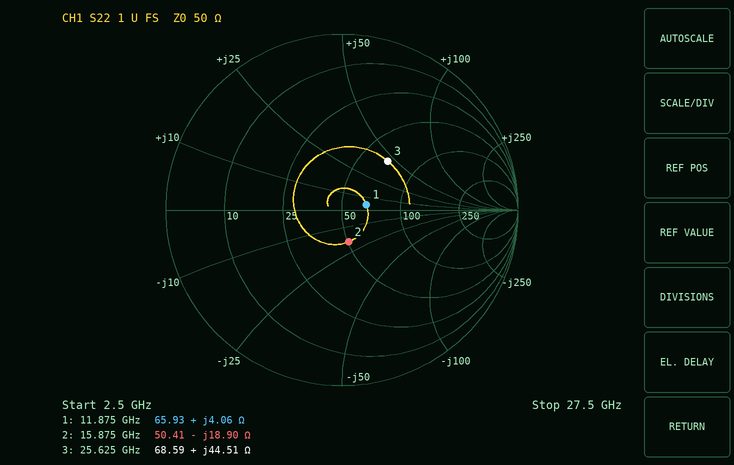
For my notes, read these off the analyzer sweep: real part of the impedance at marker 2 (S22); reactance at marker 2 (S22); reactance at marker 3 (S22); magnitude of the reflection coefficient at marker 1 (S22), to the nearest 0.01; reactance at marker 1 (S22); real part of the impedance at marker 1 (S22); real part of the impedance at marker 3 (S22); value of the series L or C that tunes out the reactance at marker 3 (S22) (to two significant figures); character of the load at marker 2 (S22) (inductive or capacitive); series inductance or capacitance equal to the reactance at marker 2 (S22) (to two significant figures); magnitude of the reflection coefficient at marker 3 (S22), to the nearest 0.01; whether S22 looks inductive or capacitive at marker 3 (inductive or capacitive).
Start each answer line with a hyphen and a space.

- 50.41 Ω
- -18.90 Ω
- +44.51 Ω
- 0.14
- +4.06 Ω
- 65.93 Ω
- 68.59 Ω
- 140 fF
- capacitive
- 530 fF
- 0.38
- inductive
